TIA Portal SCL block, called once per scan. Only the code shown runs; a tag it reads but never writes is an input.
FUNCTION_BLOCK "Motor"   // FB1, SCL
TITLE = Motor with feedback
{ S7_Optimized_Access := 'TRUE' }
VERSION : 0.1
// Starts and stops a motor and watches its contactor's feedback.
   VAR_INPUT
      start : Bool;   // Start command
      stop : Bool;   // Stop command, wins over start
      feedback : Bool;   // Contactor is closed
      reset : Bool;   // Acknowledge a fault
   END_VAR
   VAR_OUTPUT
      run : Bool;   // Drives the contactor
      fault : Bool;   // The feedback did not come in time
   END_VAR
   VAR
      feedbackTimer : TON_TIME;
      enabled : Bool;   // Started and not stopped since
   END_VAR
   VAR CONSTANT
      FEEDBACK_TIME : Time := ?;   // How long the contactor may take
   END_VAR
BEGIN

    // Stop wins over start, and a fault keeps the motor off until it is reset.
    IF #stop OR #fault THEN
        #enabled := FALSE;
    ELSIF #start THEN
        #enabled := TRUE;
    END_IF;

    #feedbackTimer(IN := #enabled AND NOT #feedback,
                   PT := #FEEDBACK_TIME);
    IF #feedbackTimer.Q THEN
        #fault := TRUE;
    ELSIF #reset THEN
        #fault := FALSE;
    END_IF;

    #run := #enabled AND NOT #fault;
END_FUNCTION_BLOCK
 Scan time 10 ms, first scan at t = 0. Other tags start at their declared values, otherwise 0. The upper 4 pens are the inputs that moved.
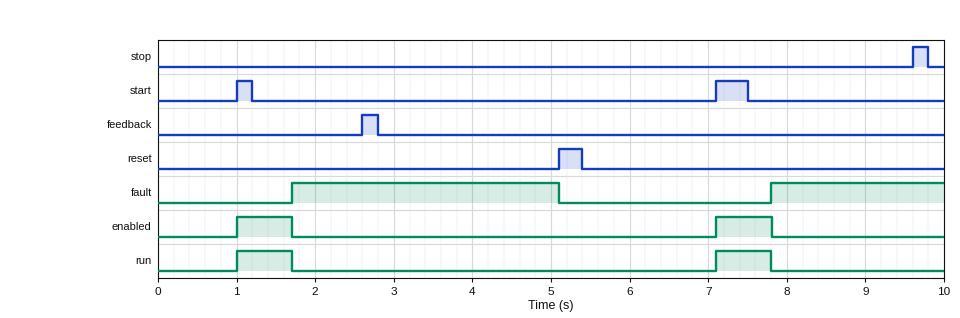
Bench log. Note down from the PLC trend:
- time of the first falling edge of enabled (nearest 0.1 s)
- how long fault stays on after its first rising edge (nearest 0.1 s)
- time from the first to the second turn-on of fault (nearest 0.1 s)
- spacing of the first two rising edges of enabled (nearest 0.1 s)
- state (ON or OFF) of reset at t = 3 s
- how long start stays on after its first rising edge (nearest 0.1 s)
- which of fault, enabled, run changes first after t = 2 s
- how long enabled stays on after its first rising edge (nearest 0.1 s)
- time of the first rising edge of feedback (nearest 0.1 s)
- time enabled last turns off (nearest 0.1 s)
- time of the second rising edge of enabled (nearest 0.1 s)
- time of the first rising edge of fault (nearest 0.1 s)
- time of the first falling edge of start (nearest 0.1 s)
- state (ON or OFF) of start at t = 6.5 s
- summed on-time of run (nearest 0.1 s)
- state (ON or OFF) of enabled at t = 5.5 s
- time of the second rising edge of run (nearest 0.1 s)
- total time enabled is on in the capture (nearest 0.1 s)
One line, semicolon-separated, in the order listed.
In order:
1.7 s; 3.4 s; 6.1 s; 6.1 s; OFF; 0.2 s; fault; 0.7 s; 2.6 s; 7.8 s; 7.1 s; 1.7 s; 1.2 s; OFF; 1.4 s; OFF; 7.1 s; 1.4 s
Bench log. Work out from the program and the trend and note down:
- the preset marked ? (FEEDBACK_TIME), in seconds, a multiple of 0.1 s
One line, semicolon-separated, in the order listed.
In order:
0.7 s
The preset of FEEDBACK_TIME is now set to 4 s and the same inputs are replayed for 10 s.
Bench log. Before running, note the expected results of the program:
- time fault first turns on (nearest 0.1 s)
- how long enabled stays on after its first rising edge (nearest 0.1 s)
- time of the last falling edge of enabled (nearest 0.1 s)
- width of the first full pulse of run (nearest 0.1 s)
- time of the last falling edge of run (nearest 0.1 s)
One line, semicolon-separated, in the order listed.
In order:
6.8 s; 5.8 s; 6.8 s; 5.8 s; 6.8 s
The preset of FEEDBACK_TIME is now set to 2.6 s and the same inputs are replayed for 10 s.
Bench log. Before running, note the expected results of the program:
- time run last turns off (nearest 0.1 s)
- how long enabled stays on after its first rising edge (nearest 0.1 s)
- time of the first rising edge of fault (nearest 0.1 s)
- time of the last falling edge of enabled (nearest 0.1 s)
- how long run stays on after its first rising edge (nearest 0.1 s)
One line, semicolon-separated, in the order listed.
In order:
5.4 s; 4.4 s; 5.4 s; 5.4 s; 4.4 s
